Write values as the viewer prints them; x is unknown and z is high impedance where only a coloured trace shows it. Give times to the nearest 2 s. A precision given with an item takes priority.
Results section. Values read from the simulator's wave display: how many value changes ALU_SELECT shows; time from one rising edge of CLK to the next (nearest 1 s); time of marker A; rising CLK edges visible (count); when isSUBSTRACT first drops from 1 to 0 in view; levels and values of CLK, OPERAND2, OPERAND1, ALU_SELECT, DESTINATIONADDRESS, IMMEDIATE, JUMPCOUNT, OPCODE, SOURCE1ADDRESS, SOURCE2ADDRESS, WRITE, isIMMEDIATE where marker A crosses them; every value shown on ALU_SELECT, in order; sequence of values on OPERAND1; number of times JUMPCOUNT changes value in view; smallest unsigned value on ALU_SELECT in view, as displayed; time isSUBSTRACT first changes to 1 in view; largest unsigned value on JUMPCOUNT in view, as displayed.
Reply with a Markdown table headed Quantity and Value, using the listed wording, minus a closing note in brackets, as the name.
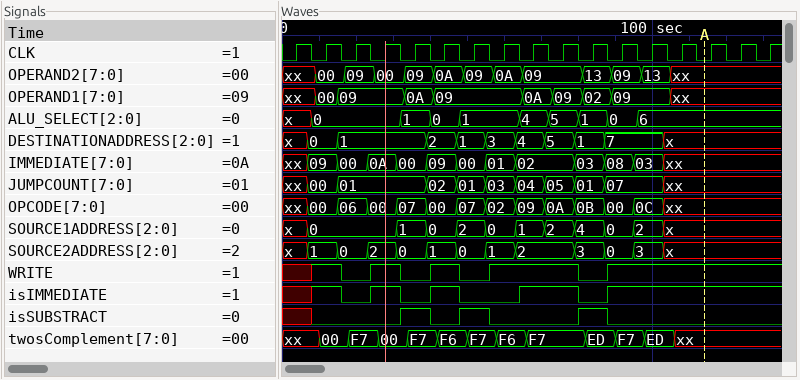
| Quantity | Value |
|---|---|
| how many value changes ALU_SELECT shows | 9 |
| time from one rising edge of CLK to the next | 8 s |
| time of marker A | 114 s |
| rising CLK edges visible | 17 |
| when isSUBSTRACT first drops from 1 to 0 in view | 40 s |
| levels and values of CLK, OPERAND2, OPERAND1, ALU_SELECT, DESTINATIONADDRESS, IMMEDIATE, JUMPCOUNT, OPCODE, SOURCE1ADDRESS, SOURCE2ADDRESS, WRITE, isIMMEDIATE where marker A crosses them | CLK=0, OPERAND2=xx, OPERAND1=xx, ALU_SELECT=6, DESTINATIONADDRESS=x, IMMEDIATE=xx, JUMPCOUNT=xx, OPCODE=xx, SOURCE1ADDRESS=x, SOURCE2ADDRESS=x, WRITE=1, isIMMEDIATE=1 |
| every value shown on ALU_SELECT, in order | x, 0, 1, 0, 1, 4, 5, 1, 0, 6 |
| sequence of values on OPERAND1 | xx, 00, 09, 0A, 09, 0A, 09, 02, 09, xx |
| number of times JUMPCOUNT changes value in view | 10 |
| smallest unsigned value on ALU_SELECT in view, as displayed | 0 |
| time isSUBSTRACT first changes to 1 in view | 32 s |
| largest unsigned value on JUMPCOUNT in view, as displayed | 07 |
